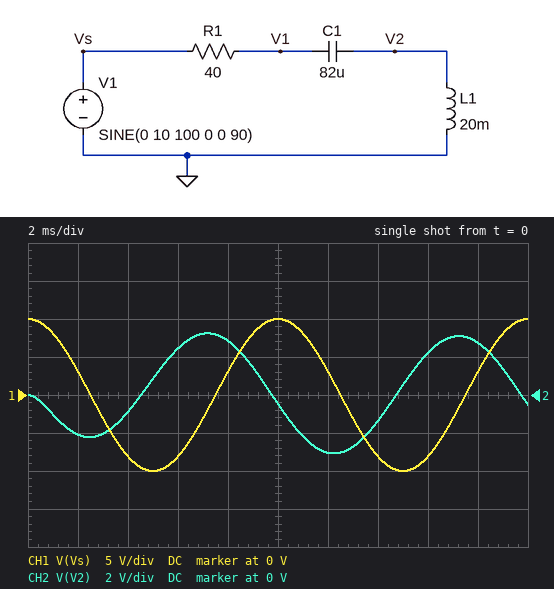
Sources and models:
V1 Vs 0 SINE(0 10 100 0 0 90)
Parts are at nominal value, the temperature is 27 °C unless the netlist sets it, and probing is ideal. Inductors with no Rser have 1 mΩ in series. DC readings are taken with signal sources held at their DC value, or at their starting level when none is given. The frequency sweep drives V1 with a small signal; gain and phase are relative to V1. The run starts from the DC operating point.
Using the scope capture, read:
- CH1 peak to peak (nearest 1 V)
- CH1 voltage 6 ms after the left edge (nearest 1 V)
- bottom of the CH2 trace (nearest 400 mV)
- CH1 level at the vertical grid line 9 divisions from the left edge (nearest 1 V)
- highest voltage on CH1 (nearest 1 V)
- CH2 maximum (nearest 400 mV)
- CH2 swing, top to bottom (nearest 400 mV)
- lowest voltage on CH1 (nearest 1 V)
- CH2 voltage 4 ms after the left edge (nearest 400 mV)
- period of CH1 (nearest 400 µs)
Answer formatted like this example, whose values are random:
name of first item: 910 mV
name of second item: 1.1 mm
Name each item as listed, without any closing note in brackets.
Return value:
CH1 peak to peak: 20 V
CH1 voltage 6 ms after the left edge: -8 V
bottom of the CH2 trace: -3.2 V
CH1 level at the vertical grid line 9 divisions from the left edge: 3 V
highest voltage on CH1: 10 V
CH2 maximum: 3.2 V
CH2 swing, top to bottom: 6.4 V
lowest voltage on CH1: -10 V
CH2 voltage 4 ms after the left edge: -800 mV
period of CH1: 10.0 ms
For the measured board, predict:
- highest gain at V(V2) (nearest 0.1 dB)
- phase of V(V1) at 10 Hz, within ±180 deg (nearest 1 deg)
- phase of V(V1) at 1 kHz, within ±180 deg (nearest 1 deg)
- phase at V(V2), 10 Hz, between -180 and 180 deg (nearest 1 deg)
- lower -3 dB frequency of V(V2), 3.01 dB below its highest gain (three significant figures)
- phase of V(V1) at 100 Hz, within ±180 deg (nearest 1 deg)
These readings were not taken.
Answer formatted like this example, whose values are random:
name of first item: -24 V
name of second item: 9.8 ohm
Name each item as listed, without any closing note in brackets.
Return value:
highest gain at V(V2): 0 dB
phase of V(V1) at 10 Hz, within ±180 deg: -12 deg
phase of V(V1) at 1 kHz, within ±180 deg: 18 deg
phase at V(V2), 10 Hz, between -180 and 180 deg: 168 deg
lower -3 dB frequency of V(V2), 3.01 dB below its highest gain: 271 Hz
phase of V(V1) at 100 Hz, within ±180 deg: -80 deg
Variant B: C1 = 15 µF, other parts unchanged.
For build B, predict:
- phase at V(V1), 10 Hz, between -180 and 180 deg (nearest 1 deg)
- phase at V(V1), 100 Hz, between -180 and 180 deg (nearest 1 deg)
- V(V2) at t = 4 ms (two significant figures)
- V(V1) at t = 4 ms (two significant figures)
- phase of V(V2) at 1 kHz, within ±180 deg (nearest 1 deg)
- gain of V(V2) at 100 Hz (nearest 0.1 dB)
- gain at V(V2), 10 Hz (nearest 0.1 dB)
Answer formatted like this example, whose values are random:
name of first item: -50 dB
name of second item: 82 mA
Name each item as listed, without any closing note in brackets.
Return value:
phase at V(V1), 10 Hz, between -180 and 180 deg: -2 deg
phase at V(V1), 100 Hz, between -180 and 180 deg: -23 deg
V(V2) at t = 4 ms: 650 mV
V(V1) at t = 4 ms: -4.7 V
phase of V(V2) at 1 kHz, within ±180 deg: 19 deg
gain of V(V2) at 100 Hz: -18.2 dB
gain at V(V2), 10 Hz: -58.5 dB
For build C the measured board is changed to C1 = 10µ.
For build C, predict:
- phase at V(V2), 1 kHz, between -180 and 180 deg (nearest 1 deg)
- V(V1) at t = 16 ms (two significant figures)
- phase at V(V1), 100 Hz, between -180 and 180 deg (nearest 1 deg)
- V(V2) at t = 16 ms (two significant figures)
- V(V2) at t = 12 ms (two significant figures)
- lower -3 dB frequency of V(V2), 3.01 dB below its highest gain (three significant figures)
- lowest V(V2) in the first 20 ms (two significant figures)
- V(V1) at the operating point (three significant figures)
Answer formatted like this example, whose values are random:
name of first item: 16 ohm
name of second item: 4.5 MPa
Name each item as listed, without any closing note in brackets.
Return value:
phase at V(V2), 1 kHz, between -180 and 180 deg: 20 deg
V(V1) at t = 16 ms: -9.0 V
phase at V(V1), 100 Hz, between -180 and 180 deg: -15 deg
V(V2) at t = 16 ms: 770 mV
V(V2) at t = 12 ms: -450 mV
lower -3 dB frequency of V(V2), 3.01 dB below its highest gain: 301 Hz
lowest V(V2) in the first 20 ms: -830 mV
V(V1) at the operating point: 10.0 V
